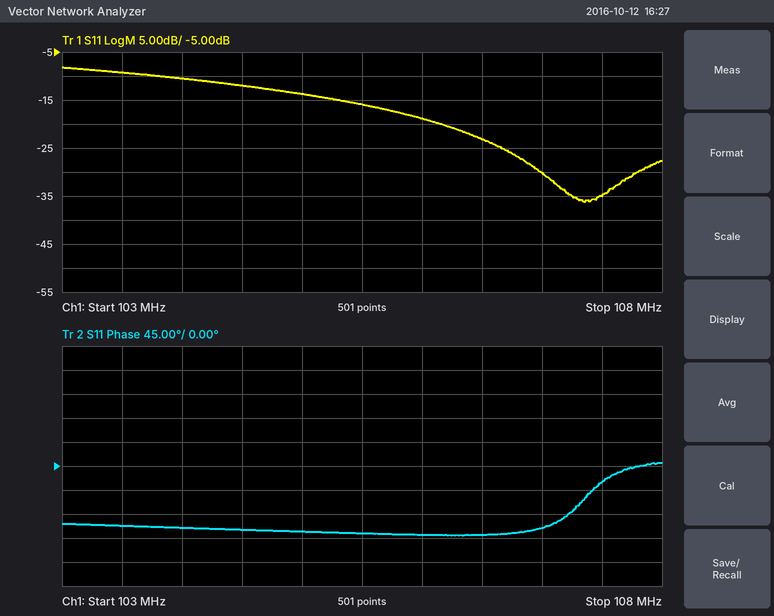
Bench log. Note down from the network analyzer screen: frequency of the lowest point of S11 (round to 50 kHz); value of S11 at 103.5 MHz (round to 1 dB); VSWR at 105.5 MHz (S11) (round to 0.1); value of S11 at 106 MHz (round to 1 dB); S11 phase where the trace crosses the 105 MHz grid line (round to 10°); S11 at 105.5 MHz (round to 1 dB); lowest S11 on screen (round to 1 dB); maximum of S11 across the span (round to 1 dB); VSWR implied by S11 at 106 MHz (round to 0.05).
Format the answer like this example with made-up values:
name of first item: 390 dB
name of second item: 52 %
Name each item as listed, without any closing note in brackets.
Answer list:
frequency of the lowest point of S11: 107.35 MHz
value of S11 at 103.5 MHz: -9 dB
VSWR at 105.5 MHz (S11): 1.4
value of S11 at 106 MHz: -19 dB
S11 phase where the trace crosses the 105 MHz grid line: -120°
S11 at 105.5 MHz: -16 dB
lowest S11 on screen: -36 dB
maximum of S11 across the span: -8 dB
VSWR implied by S11 at 106 MHz: 1.25
